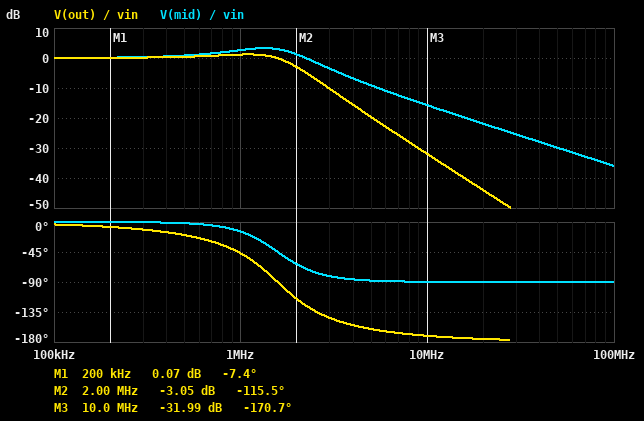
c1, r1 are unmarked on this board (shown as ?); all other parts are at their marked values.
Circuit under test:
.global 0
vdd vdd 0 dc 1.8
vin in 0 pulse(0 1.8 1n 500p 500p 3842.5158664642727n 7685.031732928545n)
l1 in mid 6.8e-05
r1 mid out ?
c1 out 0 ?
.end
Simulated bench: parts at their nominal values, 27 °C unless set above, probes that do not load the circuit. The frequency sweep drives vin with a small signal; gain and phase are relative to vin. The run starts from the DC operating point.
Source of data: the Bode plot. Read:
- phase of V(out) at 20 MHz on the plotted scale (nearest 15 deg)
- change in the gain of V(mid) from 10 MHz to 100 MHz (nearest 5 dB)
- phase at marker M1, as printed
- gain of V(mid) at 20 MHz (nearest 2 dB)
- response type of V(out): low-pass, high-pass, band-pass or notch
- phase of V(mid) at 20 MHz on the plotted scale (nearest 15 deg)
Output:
-180 deg
-20 dB
-7.4 deg
-22 dB
low-pass
-90 deg
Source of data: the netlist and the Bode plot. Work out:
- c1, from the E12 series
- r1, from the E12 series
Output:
150 pF
680 Ω
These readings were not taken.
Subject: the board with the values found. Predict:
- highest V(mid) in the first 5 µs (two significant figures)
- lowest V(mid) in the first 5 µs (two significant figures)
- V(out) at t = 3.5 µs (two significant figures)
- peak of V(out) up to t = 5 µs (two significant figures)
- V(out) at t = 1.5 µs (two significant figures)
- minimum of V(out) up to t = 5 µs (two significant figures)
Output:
2.3 V
-530 mV
1.8 V
2.1 V
1.8 V
-290 mV
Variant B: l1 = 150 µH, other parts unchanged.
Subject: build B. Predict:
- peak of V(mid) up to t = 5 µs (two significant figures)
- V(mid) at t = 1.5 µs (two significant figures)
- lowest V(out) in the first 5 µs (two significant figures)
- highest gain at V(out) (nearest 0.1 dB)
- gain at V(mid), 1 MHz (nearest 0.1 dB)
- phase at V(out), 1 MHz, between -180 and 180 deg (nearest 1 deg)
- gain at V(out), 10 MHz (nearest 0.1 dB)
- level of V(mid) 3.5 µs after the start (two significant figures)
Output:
2.5 V
1.9 V
-580 mV
3.9 dB
5.2 dB
-80 deg
-38.9 dB
1.8 V
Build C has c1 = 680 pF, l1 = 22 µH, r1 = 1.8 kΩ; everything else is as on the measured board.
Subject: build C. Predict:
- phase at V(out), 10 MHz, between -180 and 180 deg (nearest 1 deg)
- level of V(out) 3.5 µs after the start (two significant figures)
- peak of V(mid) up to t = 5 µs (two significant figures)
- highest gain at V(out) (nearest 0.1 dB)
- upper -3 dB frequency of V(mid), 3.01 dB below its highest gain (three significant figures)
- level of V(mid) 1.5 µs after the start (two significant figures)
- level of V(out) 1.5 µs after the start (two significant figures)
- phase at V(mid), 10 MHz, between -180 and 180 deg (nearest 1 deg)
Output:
-127 deg
1.7 V
1.8 V
0 dB
12.9 MHz
1.8 V
1.3 V
-38 deg
